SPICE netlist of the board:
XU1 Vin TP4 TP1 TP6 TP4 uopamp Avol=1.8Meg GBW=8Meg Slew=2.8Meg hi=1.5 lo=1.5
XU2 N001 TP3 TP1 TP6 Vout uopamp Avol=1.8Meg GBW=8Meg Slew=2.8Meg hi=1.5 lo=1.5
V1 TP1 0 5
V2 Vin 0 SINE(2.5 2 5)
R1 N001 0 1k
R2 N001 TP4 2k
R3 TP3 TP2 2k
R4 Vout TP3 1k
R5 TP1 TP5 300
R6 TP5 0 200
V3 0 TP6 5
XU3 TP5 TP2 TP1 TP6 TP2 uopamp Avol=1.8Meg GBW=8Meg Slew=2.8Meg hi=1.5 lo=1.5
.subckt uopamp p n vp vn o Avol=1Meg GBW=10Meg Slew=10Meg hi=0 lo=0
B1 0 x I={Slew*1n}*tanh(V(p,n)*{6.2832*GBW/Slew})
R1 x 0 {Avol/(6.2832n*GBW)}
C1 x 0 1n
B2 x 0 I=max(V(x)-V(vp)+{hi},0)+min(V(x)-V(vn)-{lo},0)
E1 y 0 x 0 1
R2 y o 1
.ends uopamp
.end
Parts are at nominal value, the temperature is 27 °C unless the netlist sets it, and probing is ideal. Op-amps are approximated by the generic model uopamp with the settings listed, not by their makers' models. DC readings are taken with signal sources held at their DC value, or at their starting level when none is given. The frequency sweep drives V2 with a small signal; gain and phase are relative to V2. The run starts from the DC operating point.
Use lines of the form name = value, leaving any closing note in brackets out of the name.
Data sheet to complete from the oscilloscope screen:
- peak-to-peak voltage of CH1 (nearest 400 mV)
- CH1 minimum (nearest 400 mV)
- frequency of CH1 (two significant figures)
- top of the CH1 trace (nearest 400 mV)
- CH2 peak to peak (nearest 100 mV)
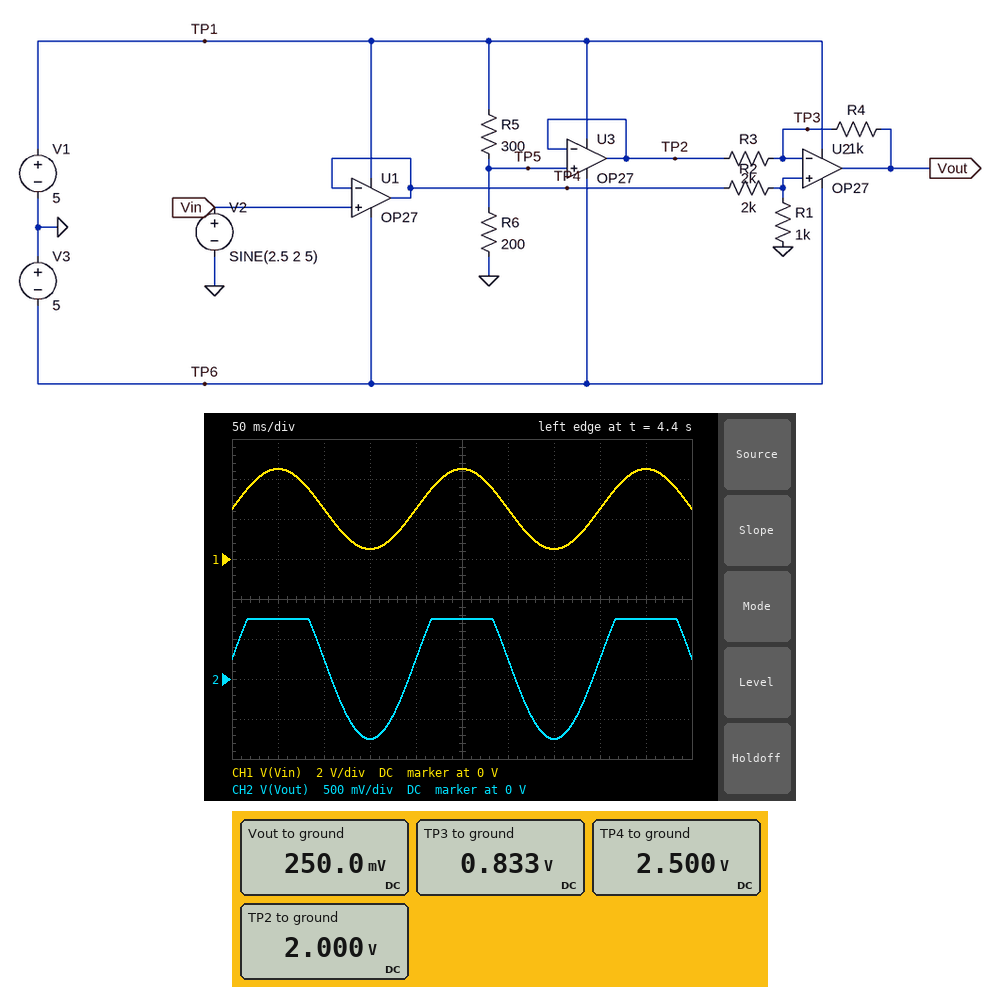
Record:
peak-to-peak voltage of CH1 = 4.0 V
CH1 minimum = 400 mV
frequency of CH1 = 5.0 Hz
top of the CH1 trace = 4.4 V
CH2 peak to peak = 1.5 V
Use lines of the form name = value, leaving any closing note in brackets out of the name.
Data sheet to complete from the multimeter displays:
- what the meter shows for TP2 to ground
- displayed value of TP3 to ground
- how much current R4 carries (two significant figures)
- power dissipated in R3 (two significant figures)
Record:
what the meter shows for TP2 to ground = 2.000 V
displayed value of TP3 to ground = 0.833 V
how much current R4 carries = 580 µA
power dissipated in R3 = 680 µW
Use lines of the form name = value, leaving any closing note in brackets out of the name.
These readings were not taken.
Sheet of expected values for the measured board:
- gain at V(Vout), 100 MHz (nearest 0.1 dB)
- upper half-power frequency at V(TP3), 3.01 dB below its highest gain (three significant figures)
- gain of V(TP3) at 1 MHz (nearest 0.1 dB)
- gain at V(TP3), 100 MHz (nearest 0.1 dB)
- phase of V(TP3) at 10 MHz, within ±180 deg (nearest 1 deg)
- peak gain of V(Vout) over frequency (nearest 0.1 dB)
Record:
gain at V(Vout), 100 MHz = -53.5 dB
upper half-power frequency at V(TP3), 3.01 dB below its highest gain = 4.08 MHz
gain of V(TP3) at 1 MHz = -9.8 dB
gain at V(TP3), 100 MHz = -57.0 dB
phase of V(TP3) at 10 MHz, within ±180 deg = -113 deg
peak gain of V(Vout) over frequency = -6.0 dB
